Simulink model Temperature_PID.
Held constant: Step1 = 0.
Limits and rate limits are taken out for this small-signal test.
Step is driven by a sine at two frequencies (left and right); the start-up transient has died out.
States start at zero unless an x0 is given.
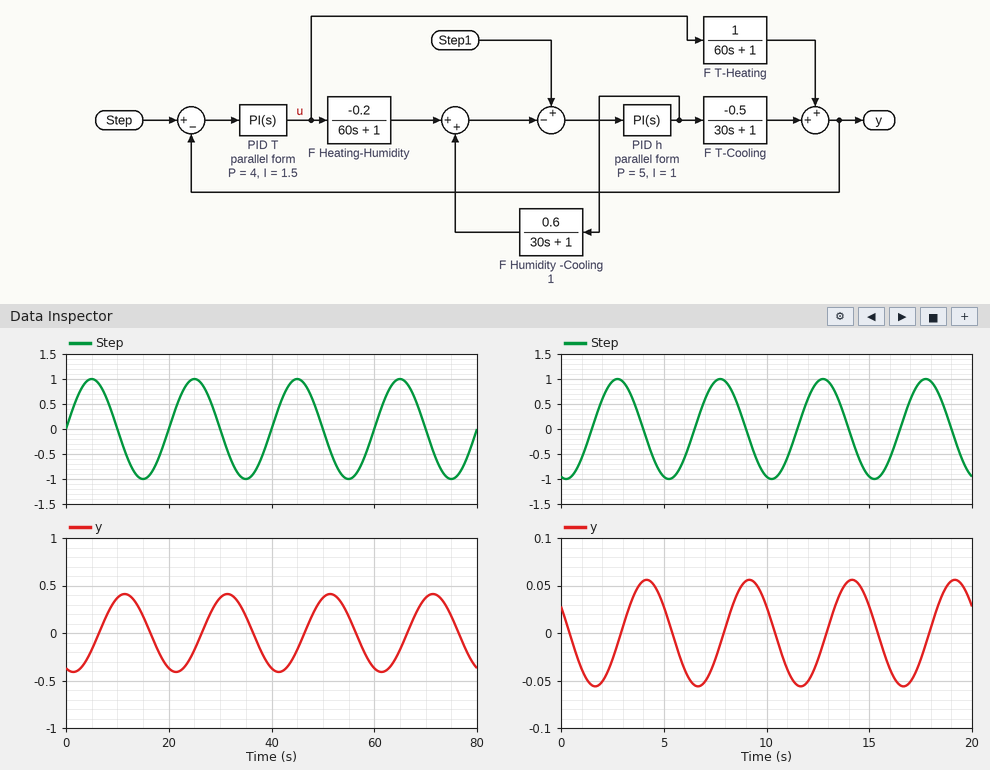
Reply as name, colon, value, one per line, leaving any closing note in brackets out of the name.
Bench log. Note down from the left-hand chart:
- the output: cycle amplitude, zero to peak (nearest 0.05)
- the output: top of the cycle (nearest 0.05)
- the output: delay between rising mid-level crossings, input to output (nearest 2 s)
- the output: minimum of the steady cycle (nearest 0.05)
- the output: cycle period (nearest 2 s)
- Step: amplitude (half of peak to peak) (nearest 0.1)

the output: cycle amplitude, zero to peak: 0.40
the output: top of the cycle: 0.40
the output: delay between rising mid-level crossings, input to output: 6 s
the output: minimum of the steady cycle: -0.40
the output: cycle period: 20 s
Step: amplitude (half of peak to peak): 1.0
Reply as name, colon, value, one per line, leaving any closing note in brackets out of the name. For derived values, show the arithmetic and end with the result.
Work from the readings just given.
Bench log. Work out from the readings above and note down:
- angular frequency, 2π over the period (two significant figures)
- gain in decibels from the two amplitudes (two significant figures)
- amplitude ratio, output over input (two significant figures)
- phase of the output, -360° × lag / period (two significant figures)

angular frequency, 2π over the period: 2π / 20 = 0.31 rad/s
gain in decibels from the two amplitudes: 20 log10(0.4 / 1) = -8.0 dB
amplitude ratio, output over input: 0.4 / 1 = 0.40
phase of the output, -360° × lag / period: -360 × 6 / 20 = -110°
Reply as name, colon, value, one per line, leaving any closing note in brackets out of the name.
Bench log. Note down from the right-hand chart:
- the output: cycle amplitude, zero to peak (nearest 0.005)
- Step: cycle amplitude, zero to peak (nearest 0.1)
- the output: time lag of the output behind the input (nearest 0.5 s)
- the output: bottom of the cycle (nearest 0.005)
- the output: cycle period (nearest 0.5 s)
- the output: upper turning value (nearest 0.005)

the output: cycle amplitude, zero to peak: 0.055
Step: cycle amplitude, zero to peak: 1.0
the output: time lag of the output behind the input: 1.5 s
the output: bottom of the cycle: -0.055
the output: cycle period: 5.0 s
the output: upper turning value: 0.055
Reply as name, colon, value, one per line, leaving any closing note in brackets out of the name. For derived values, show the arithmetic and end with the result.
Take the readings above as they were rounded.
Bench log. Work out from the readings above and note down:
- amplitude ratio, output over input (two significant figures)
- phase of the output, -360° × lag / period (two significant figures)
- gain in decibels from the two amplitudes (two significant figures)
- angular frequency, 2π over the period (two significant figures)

amplitude ratio, output over input: 0.055 / 1 = 0.055
phase of the output, -360° × lag / period: -360 × 1.5 / 5 = -110°
gain in decibels from the two amplitudes: 20 log10(0.055 / 1) = -25 dB
angular frequency, 2π over the period: 2π / 5 = 1.3 rad/s
